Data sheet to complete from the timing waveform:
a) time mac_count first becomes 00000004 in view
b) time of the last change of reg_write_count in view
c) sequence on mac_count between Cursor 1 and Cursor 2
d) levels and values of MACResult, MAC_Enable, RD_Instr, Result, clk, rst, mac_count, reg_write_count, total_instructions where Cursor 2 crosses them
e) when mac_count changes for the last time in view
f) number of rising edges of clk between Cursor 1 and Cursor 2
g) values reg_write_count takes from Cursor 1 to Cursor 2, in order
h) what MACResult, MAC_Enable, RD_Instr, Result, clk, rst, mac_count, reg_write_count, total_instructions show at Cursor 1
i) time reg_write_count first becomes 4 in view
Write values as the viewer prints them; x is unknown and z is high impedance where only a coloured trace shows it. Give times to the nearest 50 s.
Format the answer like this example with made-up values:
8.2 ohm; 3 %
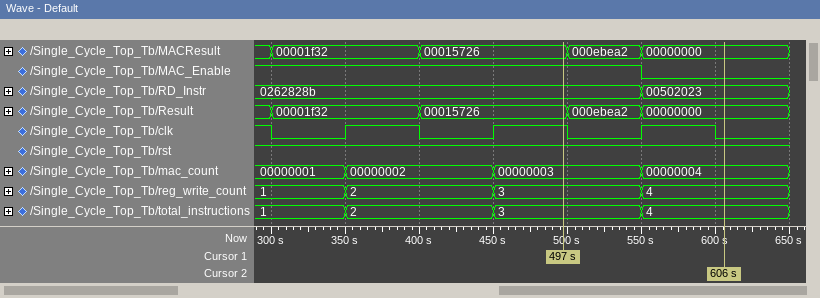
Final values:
550 s; 550 s; 00000003, 00000004; MACResult=00000000, MAC_Enable=0, RD_Instr=00502023, Result=00000000, clk=0, rst=1, mac_count=00000004, reg_write_count=4, total_instructions=4; 550 s; 1; 3, 4; MACResult=00015726, MAC_Enable=1, RD_Instr=0262828b, Result=00015726, clk=1, rst=1, mac_count=00000003, reg_write_count=3, total_instructions=3; 550 s
